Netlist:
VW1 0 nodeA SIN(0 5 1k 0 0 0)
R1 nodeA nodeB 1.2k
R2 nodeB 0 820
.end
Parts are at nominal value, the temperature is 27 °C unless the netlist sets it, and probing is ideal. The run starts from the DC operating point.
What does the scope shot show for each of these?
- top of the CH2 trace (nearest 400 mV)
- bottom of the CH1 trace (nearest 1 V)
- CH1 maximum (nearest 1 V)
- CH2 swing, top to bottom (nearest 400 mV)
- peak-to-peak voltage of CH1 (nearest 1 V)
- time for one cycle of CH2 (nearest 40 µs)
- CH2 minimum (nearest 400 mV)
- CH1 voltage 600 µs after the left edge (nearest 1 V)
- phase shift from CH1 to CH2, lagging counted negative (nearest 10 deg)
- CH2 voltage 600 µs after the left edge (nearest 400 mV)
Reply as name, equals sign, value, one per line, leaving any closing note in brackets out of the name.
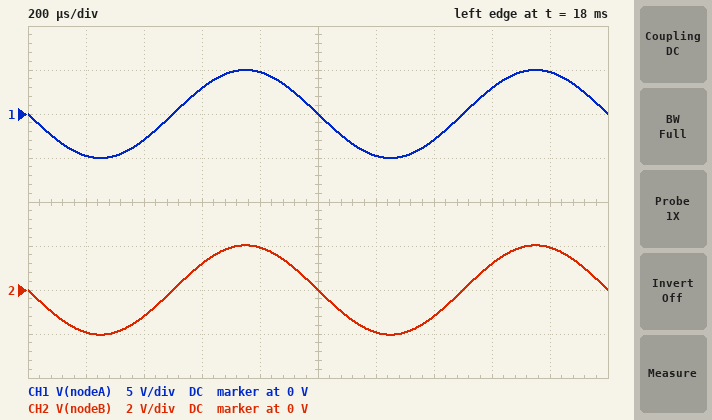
top of the CH2 trace = 2.0 V
bottom of the CH1 trace = -5 V
CH1 maximum = 5 V
CH2 swing, top to bottom = 4.0 V
peak-to-peak voltage of CH1 = 10 V
time for one cycle of CH2 = 1.00 ms
CH2 minimum = -2.0 V
CH1 voltage 600 µs after the left edge = 3 V
phase shift from CH1 to CH2, lagging counted negative = 0 deg
CH2 voltage 600 µs after the left edge = 1.2 V
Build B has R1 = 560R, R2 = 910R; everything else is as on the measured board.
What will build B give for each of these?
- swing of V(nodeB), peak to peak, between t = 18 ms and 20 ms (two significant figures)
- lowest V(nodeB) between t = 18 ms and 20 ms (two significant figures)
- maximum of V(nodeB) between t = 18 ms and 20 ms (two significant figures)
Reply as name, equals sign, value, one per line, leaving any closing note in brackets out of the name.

swing of V(nodeB), peak to peak, between t = 18 ms and 20 ms = 6.2 V
lowest V(nodeB) between t = 18 ms and 20 ms = -3.1 V
maximum of V(nodeB) between t = 18 ms and 20 ms = 3.1 V
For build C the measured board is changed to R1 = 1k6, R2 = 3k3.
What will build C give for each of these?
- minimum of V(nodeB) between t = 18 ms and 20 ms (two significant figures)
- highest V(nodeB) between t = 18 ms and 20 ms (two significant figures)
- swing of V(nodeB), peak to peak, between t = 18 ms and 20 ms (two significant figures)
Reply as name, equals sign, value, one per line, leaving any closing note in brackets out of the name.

minimum of V(nodeB) between t = 18 ms and 20 ms = -3.4 V
highest V(nodeB) between t = 18 ms and 20 ms = 3.4 V
swing of V(nodeB), peak to peak, between t = 18 ms and 20 ms = 6.7 V
